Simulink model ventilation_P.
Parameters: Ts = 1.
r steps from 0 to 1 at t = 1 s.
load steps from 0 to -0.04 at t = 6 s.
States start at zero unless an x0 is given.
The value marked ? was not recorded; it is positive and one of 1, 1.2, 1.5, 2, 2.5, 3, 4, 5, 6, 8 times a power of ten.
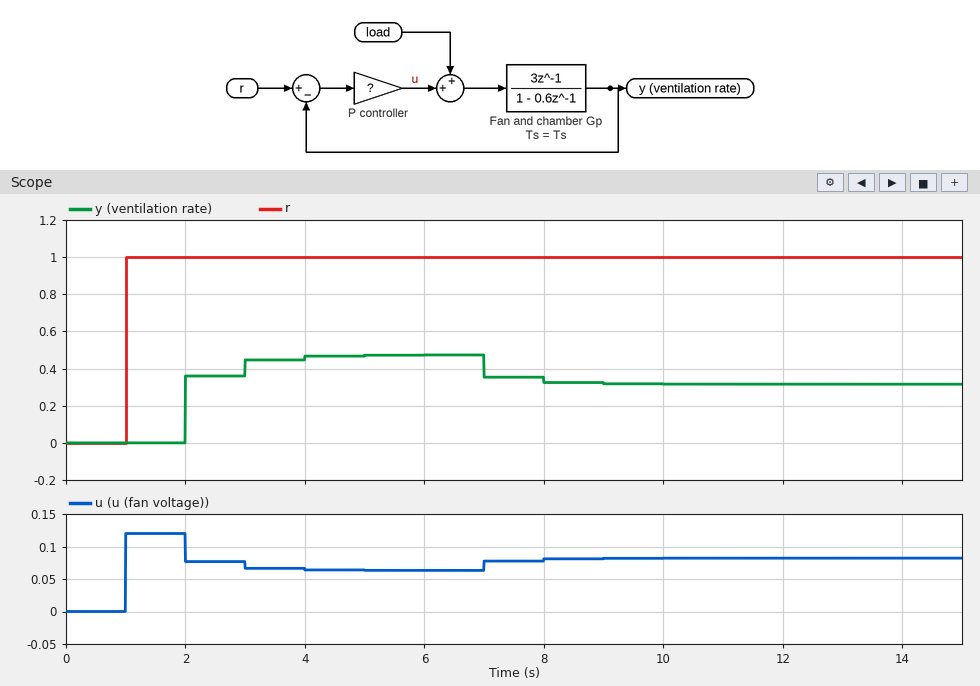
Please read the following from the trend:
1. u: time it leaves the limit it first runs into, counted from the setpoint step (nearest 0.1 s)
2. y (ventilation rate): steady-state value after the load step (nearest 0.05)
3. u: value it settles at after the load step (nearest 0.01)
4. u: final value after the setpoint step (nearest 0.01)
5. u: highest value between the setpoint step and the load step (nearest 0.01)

1.0 s
0.30
0.08
0.06
0.12
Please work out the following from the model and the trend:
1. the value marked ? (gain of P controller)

0.12
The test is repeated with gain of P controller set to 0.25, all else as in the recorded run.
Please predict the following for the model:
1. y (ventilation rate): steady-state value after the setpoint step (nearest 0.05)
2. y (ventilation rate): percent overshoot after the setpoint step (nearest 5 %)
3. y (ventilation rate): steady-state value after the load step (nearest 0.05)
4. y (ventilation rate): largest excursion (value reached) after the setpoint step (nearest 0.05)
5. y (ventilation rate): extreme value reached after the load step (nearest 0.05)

0.65
15 %
0.55
0.75
0.55
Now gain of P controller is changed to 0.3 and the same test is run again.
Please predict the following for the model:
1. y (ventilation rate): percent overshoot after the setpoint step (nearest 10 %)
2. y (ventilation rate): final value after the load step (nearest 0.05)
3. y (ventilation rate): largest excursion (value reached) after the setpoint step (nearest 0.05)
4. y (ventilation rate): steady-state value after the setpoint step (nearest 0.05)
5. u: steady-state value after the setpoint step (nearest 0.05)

30 %
0.60
0.90
0.70
0.10
